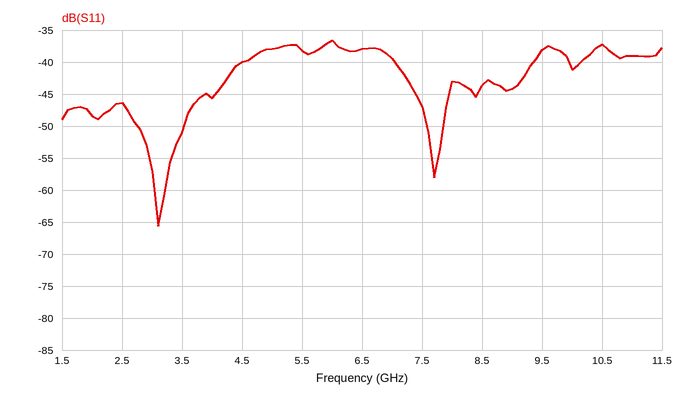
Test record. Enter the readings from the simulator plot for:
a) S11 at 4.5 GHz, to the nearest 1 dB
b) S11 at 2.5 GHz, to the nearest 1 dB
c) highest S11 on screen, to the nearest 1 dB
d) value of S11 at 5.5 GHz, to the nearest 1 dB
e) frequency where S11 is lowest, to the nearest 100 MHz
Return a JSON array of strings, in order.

["-40 dB", "-46 dB", "-37 dB", "-38 dB", "3.1 GHz"]
